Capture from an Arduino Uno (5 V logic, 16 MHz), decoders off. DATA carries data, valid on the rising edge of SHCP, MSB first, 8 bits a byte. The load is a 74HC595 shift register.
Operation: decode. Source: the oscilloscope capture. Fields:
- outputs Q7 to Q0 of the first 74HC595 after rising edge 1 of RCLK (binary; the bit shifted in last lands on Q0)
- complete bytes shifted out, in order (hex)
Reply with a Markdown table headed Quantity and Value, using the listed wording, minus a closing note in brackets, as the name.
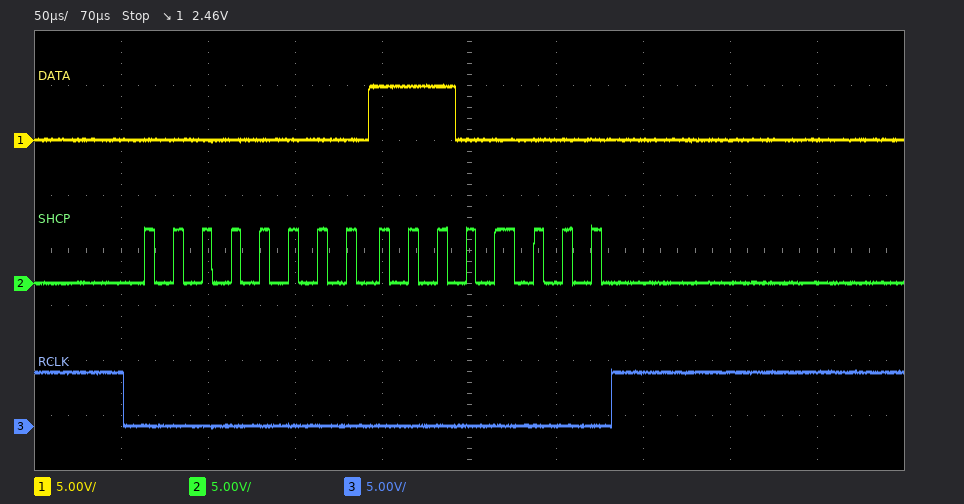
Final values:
| Quantity | Value |
|---|---|
| outputs Q7 to Q0 of the first 74HC595 after rising edge 1 of RCLK | 11100000 |
| complete bytes shifted out, in order | 0x00 0xE0 |
